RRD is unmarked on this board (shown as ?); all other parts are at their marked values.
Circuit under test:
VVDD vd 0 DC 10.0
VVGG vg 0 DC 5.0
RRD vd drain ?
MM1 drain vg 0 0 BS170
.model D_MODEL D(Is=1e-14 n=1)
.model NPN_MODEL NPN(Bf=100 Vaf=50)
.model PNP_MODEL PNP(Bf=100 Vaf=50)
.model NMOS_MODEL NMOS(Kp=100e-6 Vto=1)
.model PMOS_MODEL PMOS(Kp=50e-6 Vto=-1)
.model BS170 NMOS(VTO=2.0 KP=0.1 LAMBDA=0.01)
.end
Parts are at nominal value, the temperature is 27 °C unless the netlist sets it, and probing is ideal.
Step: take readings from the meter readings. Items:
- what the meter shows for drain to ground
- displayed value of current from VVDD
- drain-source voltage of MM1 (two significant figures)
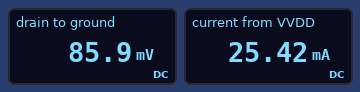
85.9 mV
25.42 mA
86 mV
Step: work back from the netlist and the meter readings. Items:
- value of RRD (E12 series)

390 Ω
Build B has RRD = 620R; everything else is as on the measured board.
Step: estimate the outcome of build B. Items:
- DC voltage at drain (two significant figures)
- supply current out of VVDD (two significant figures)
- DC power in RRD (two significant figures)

54 mV
16 mA
160 mW
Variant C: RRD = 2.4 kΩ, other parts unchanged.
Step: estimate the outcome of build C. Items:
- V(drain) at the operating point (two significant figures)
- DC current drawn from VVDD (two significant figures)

14 mV
4.2 mA
